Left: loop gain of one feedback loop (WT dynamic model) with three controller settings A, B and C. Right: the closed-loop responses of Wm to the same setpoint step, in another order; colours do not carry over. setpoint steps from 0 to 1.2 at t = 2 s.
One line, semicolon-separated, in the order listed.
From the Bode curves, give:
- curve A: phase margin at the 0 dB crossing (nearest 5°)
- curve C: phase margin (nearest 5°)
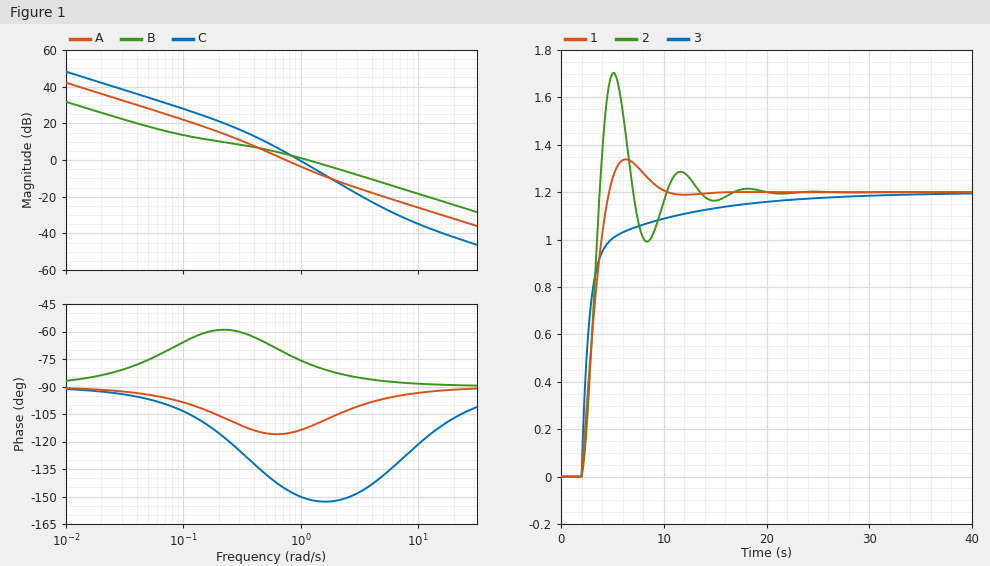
65°; 30°
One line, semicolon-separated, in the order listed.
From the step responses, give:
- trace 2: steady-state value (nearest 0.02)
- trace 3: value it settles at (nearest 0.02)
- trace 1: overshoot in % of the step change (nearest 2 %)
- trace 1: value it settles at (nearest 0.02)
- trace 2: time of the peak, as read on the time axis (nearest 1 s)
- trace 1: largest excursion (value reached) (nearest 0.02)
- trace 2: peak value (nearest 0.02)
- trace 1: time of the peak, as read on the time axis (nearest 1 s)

1.20; 1.20; 12 %; 1.20; 5 s; 1.34; 1.70; 6 s
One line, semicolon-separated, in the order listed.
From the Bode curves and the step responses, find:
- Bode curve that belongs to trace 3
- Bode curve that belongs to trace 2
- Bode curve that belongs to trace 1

B; C; A
